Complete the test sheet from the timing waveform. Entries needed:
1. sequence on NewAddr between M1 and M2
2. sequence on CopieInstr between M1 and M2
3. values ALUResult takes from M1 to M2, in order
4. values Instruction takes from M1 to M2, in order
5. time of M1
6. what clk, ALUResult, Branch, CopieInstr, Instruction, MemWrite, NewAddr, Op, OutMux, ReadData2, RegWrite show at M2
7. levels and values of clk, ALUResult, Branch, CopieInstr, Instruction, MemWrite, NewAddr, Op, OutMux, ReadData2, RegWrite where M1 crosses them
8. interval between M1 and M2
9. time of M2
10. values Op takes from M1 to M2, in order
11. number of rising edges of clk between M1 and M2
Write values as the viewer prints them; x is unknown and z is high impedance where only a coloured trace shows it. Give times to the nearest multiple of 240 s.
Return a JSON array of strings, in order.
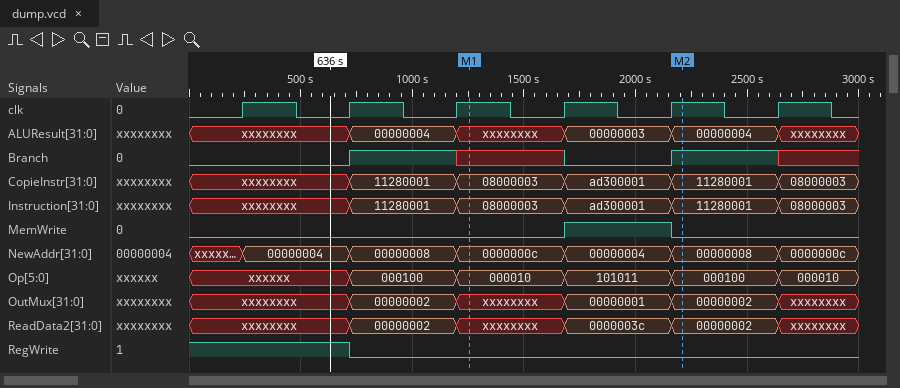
["0000000c, 00000004, 00000008", "08000003, ad300001, 11280001", "xxxxxxxx, 00000003, 00000004", "08000003, ad300001, 11280001", "1200 s", "clk=1, ALUResult=00000004, Branch=1, CopieInstr=11280001, Instruction=11280001, MemWrite=0, NewAddr=00000008, Op=000100, OutMux=00000002, ReadData2=00000002, RegWrite=0", "clk=1, ALUResult=xxxxxxxx, Branch=x, CopieInstr=08000003, Instruction=08000003, MemWrite=0, NewAddr=0000000c, Op=000010, OutMux=xxxxxxxx, ReadData2=xxxxxxxx, RegWrite=0", "960 s", "2160 s", "000010, 101011, 000100", "2"]
